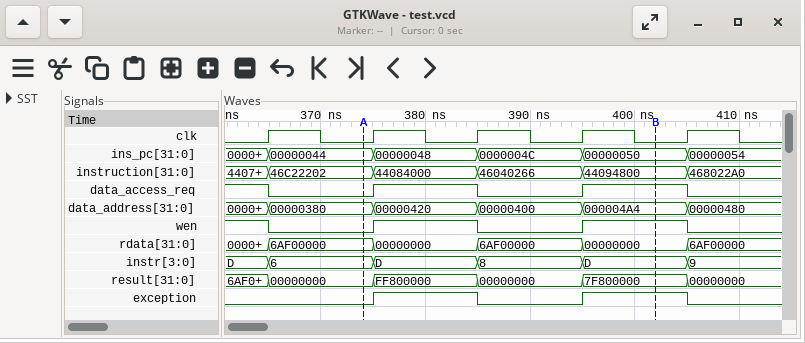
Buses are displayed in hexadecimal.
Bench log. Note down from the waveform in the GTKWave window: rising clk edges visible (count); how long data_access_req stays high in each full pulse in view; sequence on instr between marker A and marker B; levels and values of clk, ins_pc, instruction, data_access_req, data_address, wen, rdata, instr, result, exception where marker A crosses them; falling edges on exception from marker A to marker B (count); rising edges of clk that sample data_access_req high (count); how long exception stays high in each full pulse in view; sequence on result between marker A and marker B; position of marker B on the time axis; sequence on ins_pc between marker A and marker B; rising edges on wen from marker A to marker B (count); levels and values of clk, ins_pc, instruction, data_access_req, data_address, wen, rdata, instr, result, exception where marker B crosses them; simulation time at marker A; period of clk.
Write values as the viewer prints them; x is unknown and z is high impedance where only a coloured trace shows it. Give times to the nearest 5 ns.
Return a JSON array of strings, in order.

["5", "10 ns, 10 ns", "6, D, 8, D", "clk=0, ins_pc=00000044, instruction=46C22202, data_access_req=0, data_address=00000380, wen=0, rdata=6AF00000, instr=6, result=00000000, exception=0", "1", "3", "10 ns, 10 ns", "00000000, FF800000, 00000000, 7F800000", "400 ns", "00000044, 00000048, 0000004C, 00000050", "2", "clk=0, ins_pc=00000050, instruction=44094800, data_access_req=1, data_address=000004A4, wen=1, rdata=00000000, instr=D, result=7F800000, exception=1", "375 ns", "10 ns"]
